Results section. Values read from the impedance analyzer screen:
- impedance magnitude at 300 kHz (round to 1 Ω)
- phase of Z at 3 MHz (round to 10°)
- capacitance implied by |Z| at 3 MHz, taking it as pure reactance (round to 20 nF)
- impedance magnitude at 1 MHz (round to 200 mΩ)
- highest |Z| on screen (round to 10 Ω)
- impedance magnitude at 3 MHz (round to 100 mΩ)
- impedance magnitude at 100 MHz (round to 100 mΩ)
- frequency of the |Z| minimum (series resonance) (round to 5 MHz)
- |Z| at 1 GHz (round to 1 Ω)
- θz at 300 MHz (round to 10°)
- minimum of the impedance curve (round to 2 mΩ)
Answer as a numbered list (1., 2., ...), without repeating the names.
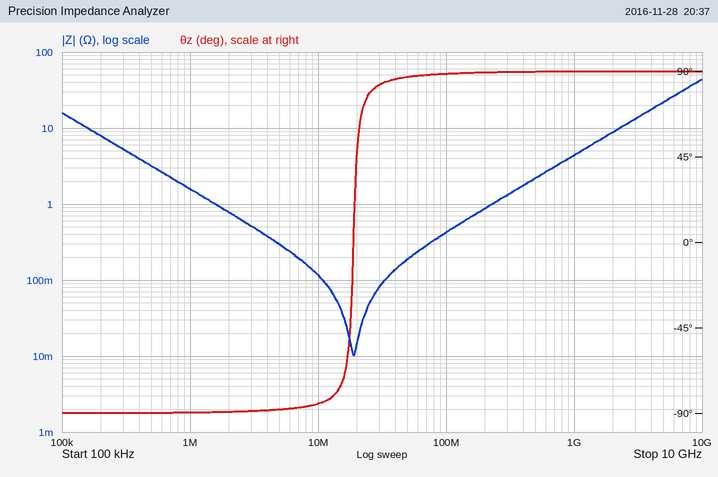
1. 5 Ω
2. -90°
3. 100 nF
4. 1.6 Ω
5. 40 Ω
6. 500 mΩ
7. 400 mΩ
8. 20 MHz
9. 4 Ω
10. 90°
11. 10 mΩ
